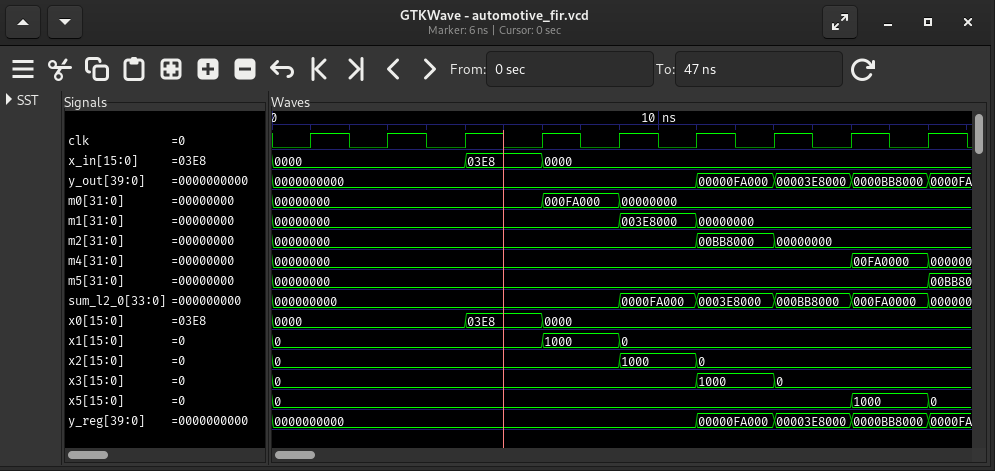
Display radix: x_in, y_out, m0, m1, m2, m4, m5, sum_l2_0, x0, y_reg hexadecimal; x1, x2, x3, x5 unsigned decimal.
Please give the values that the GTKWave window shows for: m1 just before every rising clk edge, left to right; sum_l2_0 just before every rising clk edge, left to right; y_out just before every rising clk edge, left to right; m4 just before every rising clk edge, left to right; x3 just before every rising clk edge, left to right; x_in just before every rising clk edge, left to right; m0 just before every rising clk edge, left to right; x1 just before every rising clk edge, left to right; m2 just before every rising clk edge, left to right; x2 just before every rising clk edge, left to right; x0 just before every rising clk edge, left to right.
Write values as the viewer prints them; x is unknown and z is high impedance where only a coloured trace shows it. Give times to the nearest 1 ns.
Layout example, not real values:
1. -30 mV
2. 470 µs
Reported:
1. 00000000, 00000000, 00000000, 00000000, 00000000, 003E8000, 00000000, 00000000, 00000000
2. 000000000, 000000000, 000000000, 000000000, 000000000, 0000FA000, 0003E8000, 000BB8000, 000FA0000
3. 0000000000, 0000000000, 0000000000, 0000000000, 0000000000, 0000000000, 00000FA000, 00003E8000, 0000BB8000
4. 00000000, 00000000, 00000000, 00000000, 00000000, 00000000, 00000000, 00000000, 00FA0000
5. 0, 0, 0, 0, 0, 0, 1000, 0, 0
6. 0000, 0000, 0000, 03E8, 0000, 0000, 0000, 0000, 0000
7. 00000000, 00000000, 00000000, 00000000, 000FA000, 00000000, 00000000, 00000000, 00000000
8. 0, 0, 0, 0, 1000, 0, 0, 0, 0
9. 00000000, 00000000, 00000000, 00000000, 00000000, 00000000, 00BB8000, 00000000, 00000000
10. 0, 0, 0, 0, 0, 1000, 0, 0, 0
11. 0000, 0000, 0000, 03E8, 0000, 0000, 0000, 0000, 0000
